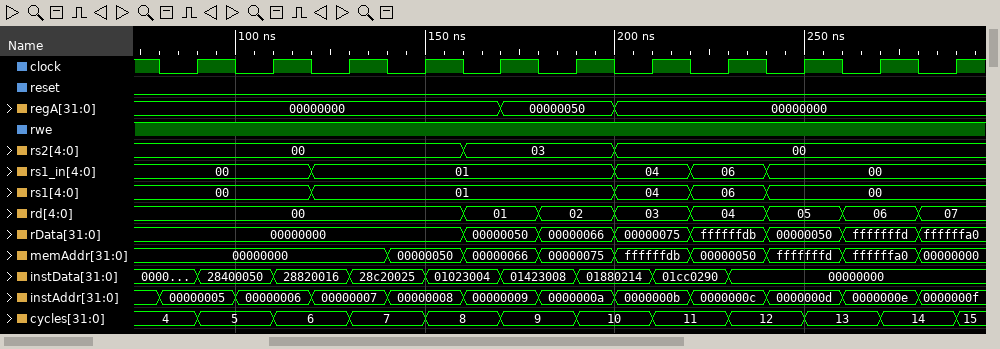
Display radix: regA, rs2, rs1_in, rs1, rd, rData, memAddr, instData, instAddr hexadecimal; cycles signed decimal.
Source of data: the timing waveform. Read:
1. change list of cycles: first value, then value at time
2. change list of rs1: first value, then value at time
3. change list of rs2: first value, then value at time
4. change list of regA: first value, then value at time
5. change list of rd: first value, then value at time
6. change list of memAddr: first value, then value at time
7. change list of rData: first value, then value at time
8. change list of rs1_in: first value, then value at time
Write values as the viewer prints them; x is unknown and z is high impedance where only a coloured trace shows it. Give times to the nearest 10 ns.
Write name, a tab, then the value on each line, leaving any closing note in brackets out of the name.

change list of cycles: first value, then value at time	4, 5 at 90 ns, 6 at 110 ns, 7 at 130 ns, 8 at 150 ns, 9 at 170 ns, 10 at 190 ns, 11 at 210 ns, 12 at 230 ns, 13 at 250 ns, 14 at 270 ns, 15 at 290 ns
change list of rs1: first value, then value at time	00, 01 at 120 ns, 04 at 200 ns, 06 at 220 ns, 00 at 240 ns
change list of rs2: first value, then value at time	00, 03 at 160 ns, 00 at 200 ns
change list of regA: first value, then value at time	00000000, 00000050 at 170 ns, 00000000 at 200 ns
change list of rd: first value, then value at time	00, 01 at 160 ns, 02 at 180 ns, 03 at 200 ns, 04 at 220 ns, 05 at 240 ns, 06 at 260 ns, 07 at 280 ns
change list of memAddr: first value, then value at time	00000000, 00000050 at 140 ns, 00000066 at 160 ns, 00000075 at 180 ns, ffffffdb at 200 ns, 00000050 at 220 ns, fffffffd at 240 ns, ffffffa0 at 260 ns, 00000000 at 280 ns
change list of rData: first value, then value at time	00000000, 00000050 at 160 ns, 00000066 at 180 ns, 00000075 at 200 ns, ffffffdb at 220 ns, 00000050 at 240 ns, fffffffd at 260 ns, ffffffa0 at 280 ns
change list of rs1_in: first value, then value at time	00, 01 at 120 ns, 04 at 200 ns, 06 at 220 ns, 00 at 240 ns
